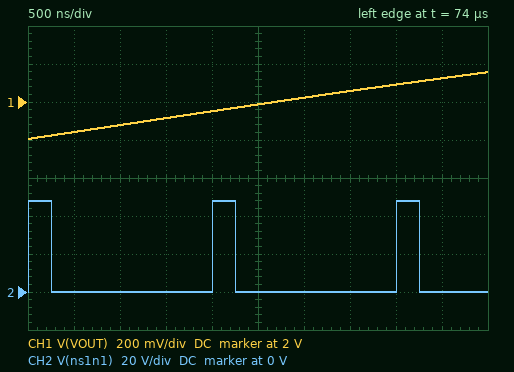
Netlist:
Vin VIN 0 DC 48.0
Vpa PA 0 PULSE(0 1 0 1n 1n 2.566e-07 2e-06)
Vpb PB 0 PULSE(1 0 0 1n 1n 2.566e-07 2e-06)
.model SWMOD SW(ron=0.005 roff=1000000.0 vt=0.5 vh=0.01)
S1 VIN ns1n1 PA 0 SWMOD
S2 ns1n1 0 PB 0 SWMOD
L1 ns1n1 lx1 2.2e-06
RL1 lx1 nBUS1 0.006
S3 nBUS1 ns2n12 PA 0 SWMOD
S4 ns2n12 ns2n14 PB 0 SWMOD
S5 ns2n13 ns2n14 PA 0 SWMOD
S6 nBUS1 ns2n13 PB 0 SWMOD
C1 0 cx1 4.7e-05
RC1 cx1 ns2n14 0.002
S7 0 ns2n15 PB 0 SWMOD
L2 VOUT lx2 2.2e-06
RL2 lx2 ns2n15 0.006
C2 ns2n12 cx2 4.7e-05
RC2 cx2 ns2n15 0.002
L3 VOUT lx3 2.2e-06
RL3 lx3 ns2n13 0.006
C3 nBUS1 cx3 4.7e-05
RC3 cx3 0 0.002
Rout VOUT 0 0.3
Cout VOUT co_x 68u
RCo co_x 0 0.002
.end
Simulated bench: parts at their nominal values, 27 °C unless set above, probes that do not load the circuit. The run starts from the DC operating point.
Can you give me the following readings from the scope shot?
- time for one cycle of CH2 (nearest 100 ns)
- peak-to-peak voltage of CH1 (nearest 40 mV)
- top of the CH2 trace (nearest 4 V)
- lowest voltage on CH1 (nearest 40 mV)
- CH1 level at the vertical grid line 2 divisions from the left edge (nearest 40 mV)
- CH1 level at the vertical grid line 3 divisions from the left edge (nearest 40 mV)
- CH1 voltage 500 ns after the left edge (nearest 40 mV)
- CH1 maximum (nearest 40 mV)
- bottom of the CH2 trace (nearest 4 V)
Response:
2.0 µs
360 mV
48 V
1.80 V
1.88 V
1.92 V
1.84 V
2.16 V
0 V
